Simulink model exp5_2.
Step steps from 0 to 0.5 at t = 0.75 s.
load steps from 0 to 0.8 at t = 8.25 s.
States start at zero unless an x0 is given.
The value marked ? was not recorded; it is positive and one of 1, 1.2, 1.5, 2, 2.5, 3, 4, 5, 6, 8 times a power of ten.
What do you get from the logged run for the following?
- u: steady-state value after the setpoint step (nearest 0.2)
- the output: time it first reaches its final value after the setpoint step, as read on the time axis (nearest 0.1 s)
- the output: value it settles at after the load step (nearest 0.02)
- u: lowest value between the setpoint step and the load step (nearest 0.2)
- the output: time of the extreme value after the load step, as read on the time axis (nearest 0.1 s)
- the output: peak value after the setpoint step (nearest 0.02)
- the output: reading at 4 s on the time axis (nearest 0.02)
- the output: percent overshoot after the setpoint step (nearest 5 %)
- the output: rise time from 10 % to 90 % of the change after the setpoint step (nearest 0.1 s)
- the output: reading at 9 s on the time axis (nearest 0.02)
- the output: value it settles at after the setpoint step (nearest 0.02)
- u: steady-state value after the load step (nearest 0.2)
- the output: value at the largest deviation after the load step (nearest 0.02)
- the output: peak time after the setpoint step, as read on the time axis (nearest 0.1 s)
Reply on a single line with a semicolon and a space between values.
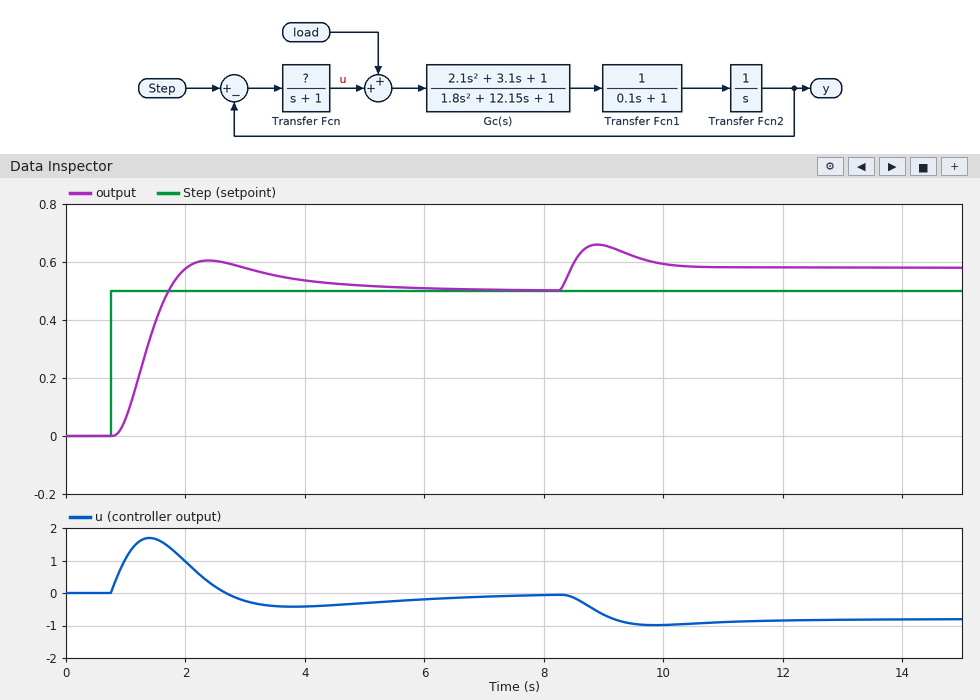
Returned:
0.0; 1.7 s; 0.58; -0.4; 8.9 s; 0.60; 0.54; 20 %; 0.6 s; 0.66; 0.50; -0.8; 0.66; 2.4 s
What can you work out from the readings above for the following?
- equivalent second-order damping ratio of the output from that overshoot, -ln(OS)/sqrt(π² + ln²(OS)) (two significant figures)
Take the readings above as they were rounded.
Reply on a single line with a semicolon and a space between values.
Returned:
0.46
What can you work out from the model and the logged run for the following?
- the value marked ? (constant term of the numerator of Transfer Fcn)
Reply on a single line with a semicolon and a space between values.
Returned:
10
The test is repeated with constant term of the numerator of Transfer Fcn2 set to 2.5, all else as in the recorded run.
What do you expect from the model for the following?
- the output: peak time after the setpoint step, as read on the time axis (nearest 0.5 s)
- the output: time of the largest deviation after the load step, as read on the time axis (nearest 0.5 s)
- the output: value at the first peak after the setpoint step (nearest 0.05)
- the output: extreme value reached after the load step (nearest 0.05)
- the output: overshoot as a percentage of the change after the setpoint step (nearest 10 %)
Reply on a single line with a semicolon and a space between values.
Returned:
1.5 s; 8.5 s; 0.70; 0.80; 40 %
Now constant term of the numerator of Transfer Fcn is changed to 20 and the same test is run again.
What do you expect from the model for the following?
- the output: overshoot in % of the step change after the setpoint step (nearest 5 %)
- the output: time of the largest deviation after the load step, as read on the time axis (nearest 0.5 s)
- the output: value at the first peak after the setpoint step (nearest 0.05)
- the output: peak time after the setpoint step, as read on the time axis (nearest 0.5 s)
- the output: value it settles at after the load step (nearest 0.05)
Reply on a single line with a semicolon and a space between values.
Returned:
35 %; 8.5 s; 0.65; 1.5 s; 0.55
